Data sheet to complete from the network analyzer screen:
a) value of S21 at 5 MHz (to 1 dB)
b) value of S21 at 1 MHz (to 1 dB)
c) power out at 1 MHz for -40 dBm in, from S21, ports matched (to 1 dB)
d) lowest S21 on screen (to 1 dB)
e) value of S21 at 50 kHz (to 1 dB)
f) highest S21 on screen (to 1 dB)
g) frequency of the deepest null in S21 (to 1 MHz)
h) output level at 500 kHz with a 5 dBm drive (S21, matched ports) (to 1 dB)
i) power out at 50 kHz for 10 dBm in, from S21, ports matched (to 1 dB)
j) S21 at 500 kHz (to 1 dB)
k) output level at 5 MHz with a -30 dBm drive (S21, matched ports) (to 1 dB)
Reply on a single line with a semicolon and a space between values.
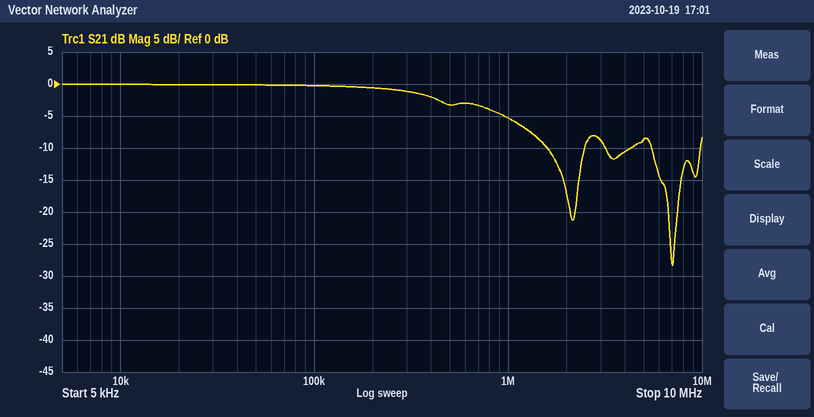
-9 dB; -5 dB; -45 dBm; -28 dB; 0 dB; 0 dB; 7 MHz; 2 dBm; 10 dBm; -3 dB; -39 dBm
